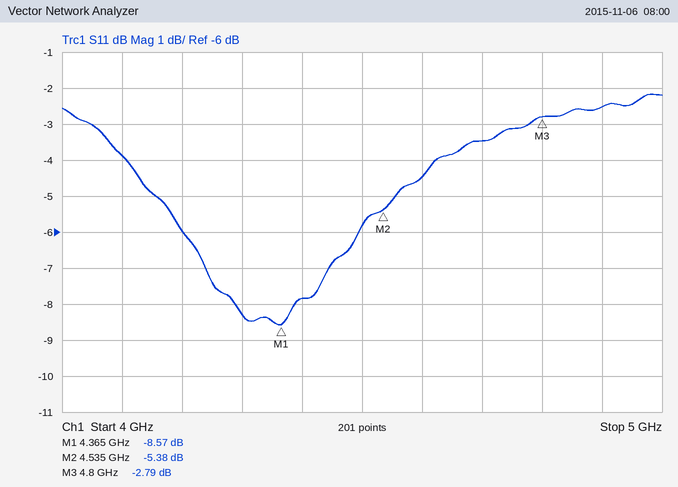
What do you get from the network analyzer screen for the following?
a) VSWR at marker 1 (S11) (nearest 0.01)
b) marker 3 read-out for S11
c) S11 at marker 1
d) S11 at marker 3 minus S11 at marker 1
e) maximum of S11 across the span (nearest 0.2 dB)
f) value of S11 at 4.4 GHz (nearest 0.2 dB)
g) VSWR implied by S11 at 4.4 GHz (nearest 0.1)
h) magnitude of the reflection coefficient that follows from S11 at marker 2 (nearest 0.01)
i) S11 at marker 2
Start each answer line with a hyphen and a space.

- 2.19
- -2.79 dB
- -8.57 dB
- 5.78 dB
- -2.2 dB
- -7.8 dB
- 2.4
- 0.54
- -5.38 dB
